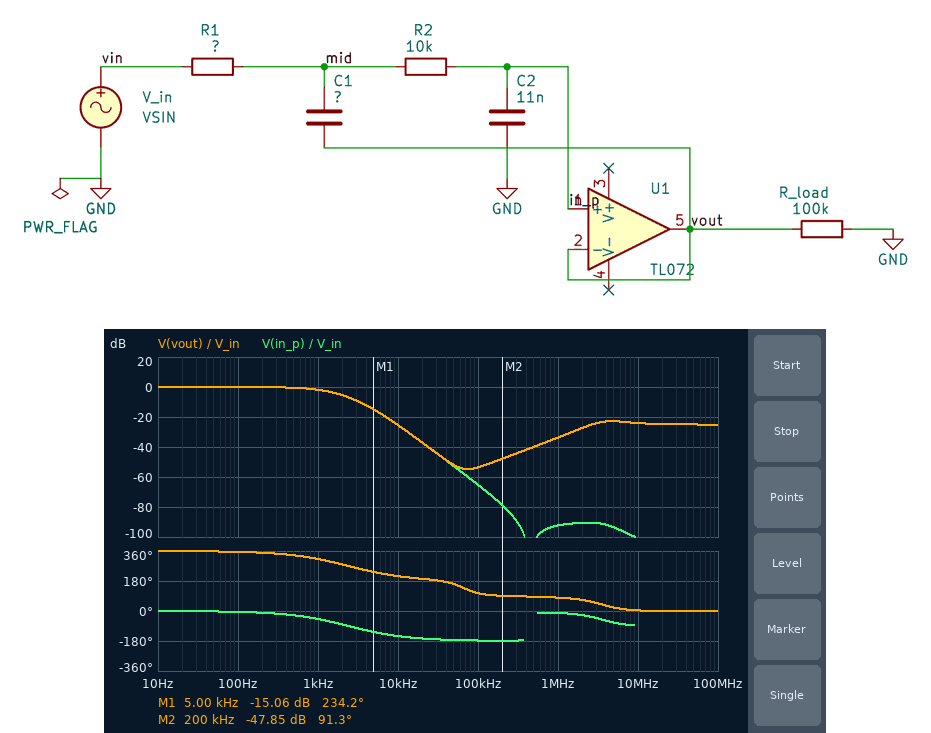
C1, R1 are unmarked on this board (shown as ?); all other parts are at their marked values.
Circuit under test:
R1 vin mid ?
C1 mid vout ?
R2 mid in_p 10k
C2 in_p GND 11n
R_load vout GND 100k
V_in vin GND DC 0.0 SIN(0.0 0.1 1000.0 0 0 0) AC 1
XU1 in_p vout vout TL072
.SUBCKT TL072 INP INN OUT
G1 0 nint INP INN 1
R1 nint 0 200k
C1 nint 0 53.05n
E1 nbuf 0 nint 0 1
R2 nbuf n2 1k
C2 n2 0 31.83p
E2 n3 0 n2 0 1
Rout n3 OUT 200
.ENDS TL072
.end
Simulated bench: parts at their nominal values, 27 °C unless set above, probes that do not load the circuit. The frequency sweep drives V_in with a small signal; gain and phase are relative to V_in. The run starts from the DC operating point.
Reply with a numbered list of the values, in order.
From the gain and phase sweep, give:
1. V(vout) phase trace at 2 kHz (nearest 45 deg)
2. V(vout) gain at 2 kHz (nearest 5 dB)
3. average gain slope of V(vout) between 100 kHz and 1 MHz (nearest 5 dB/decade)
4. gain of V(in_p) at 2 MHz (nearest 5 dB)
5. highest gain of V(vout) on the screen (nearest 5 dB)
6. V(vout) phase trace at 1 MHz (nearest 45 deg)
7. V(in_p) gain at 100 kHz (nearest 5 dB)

1. 270 deg
2. -5 dB
3. 20 dB/decade
4. -90 dB
5. 0 dB
6. 90 deg
7. -65 dB
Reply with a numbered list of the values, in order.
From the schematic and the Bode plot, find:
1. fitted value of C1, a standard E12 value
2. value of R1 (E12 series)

1. 12 nF
2. 3.3 kΩ
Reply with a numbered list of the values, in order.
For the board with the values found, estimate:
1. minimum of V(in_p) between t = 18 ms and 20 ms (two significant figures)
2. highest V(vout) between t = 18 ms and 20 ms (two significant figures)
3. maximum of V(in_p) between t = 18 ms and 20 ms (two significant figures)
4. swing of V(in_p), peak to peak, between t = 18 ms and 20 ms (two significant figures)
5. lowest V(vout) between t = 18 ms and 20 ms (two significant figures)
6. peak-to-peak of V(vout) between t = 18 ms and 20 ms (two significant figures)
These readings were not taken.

1. -81 mV
2. 81 mV
3. 81 mV
4. 160 mV
5. -81 mV
6. 160 mV
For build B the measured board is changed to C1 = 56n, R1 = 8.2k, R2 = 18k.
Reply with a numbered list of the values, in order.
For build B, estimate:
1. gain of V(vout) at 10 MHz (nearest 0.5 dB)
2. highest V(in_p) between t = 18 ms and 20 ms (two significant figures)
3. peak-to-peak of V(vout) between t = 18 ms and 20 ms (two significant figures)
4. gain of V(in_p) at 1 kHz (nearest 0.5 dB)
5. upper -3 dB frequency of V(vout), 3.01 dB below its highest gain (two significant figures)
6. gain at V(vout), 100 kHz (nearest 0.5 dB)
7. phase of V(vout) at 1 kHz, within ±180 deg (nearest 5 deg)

1. -31.5 dB
2. 32 mV
3. 63 mV
4. -10.0 dB
5. 620 Hz
6. -62.0 dB
7. -145 deg
